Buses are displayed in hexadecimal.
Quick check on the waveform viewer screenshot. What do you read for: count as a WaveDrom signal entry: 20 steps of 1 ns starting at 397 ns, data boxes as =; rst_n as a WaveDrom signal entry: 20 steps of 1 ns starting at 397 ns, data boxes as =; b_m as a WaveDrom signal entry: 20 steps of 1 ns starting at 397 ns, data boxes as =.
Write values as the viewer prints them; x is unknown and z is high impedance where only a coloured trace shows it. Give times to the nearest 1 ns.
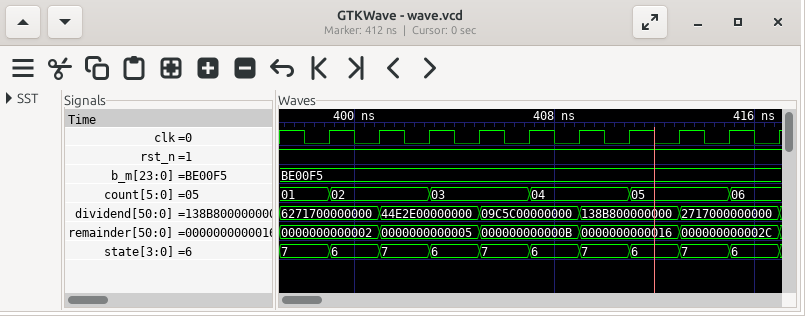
{name: 'count', wave: '=.=...=...=...=...=.', data: '01 02 03 04 05 06'}
{name: 'rst_n', wave: '1...................'}
{name: 'b_m', wave: '=...................', data: 'BE00F5'}
